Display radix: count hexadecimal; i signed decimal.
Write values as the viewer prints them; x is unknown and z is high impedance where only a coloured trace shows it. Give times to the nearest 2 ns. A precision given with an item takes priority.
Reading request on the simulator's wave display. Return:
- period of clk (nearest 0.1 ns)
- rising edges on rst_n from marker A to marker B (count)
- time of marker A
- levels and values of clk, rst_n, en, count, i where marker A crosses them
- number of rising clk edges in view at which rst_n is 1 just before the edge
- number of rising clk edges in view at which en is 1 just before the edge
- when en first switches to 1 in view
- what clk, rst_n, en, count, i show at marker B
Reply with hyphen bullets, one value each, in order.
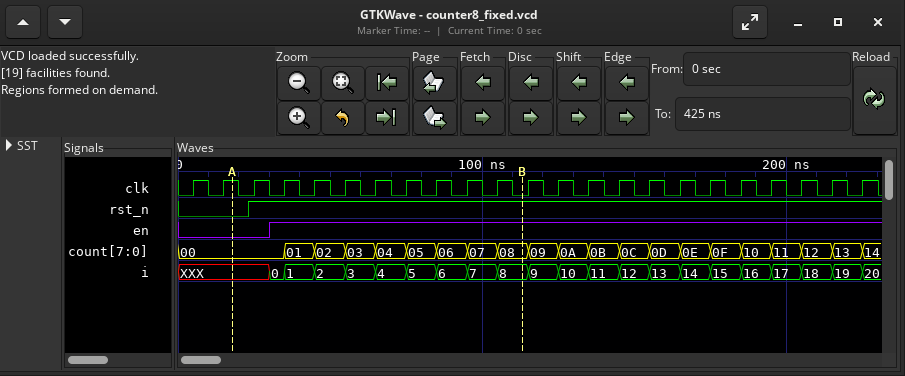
- 10 ns
- 1
- 18 ns
- clk=1, rst_n=0, en=0, count=00, i=XXX
- 21
- 20
- 30 ns
- clk=0, rst_n=1, en=1, count=08, i=8
